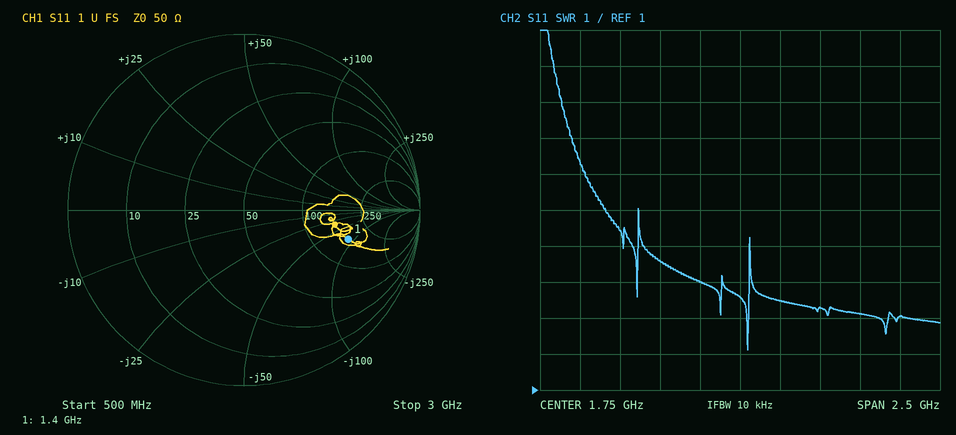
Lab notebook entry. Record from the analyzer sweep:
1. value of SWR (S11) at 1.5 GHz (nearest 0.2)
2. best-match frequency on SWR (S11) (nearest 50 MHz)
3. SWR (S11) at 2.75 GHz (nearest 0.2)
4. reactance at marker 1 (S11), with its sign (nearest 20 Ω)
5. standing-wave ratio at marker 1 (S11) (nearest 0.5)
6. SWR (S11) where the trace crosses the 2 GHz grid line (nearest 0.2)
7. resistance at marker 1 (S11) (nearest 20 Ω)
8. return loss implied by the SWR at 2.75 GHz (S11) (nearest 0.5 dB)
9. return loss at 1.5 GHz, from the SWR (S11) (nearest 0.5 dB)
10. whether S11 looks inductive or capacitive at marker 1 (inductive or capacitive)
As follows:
4.0
1.80 GHz
3.0
-80 Ω
4.0
3.4
160 Ω
6.0 dB
4.5 dB
capacitive
